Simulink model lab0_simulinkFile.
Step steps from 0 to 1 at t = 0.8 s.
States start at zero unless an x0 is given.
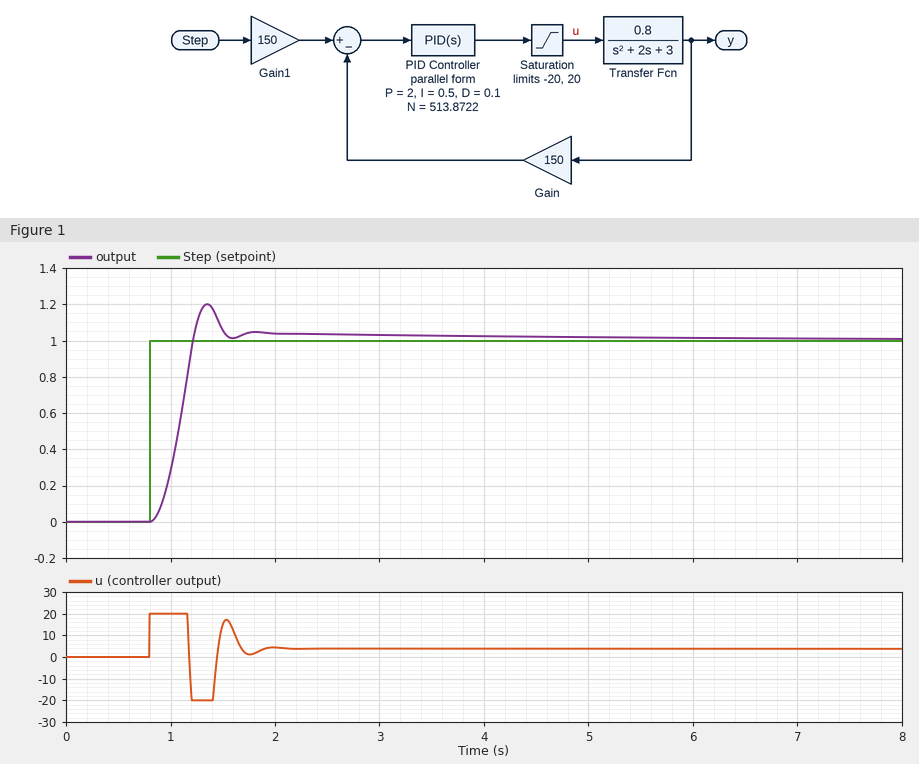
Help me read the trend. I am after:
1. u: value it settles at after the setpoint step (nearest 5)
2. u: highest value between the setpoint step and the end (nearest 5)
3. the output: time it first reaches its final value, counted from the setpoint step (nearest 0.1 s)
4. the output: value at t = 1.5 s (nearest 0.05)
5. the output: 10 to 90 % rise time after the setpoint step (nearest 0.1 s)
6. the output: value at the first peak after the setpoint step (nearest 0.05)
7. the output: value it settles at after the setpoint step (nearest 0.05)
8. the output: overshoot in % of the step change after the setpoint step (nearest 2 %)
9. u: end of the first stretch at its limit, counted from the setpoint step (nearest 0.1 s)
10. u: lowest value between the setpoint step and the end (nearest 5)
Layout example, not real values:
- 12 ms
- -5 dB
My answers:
- 5
- 20
- 0.4 s
- 1.05
- 0.3 s
- 1.20
- 1.00
- 20 %
- 0.4 s
- -20
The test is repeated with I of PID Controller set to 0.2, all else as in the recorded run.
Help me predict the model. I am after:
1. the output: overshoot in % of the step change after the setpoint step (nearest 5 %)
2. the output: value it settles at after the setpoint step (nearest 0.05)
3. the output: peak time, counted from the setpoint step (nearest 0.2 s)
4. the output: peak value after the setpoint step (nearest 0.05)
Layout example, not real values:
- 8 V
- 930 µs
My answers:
- 15 %
- 1.00
- 0.6 s
- 1.15
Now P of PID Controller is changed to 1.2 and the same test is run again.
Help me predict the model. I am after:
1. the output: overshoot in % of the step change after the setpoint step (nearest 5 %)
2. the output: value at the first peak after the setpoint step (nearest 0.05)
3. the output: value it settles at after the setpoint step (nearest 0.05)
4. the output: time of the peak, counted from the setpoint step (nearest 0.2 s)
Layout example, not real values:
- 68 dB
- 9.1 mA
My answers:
- 15 %
- 1.15
- 1.00
- 0.6 s
